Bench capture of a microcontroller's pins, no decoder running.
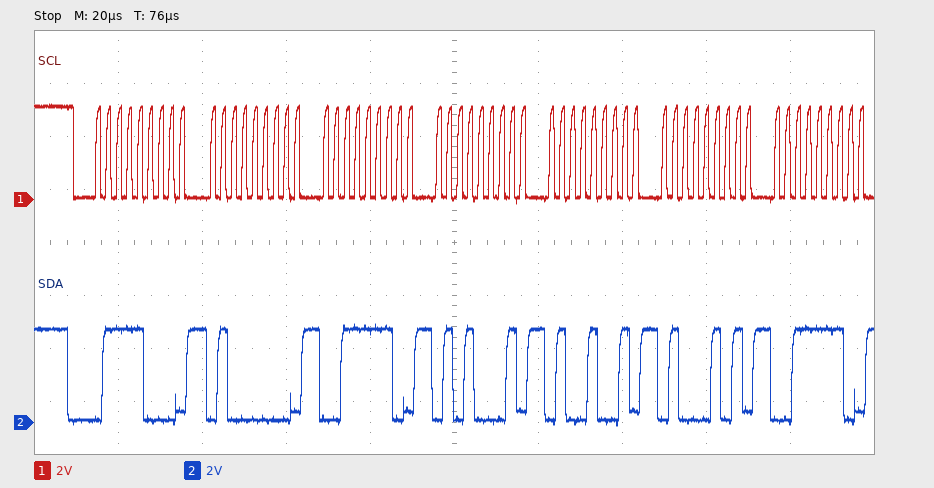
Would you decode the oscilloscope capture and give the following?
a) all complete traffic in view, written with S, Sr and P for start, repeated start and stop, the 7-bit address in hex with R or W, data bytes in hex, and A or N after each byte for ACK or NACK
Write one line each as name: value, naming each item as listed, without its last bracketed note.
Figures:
all complete traffic in view, written with S, Sr and P for start, repeated start and stop, the 7-bit address in hex with R or W, data bytes in hex, and A or N after each byte for ACK or NACK: S 3CW A 40 A 3E A 51 A 49 A 45 A 3E A
